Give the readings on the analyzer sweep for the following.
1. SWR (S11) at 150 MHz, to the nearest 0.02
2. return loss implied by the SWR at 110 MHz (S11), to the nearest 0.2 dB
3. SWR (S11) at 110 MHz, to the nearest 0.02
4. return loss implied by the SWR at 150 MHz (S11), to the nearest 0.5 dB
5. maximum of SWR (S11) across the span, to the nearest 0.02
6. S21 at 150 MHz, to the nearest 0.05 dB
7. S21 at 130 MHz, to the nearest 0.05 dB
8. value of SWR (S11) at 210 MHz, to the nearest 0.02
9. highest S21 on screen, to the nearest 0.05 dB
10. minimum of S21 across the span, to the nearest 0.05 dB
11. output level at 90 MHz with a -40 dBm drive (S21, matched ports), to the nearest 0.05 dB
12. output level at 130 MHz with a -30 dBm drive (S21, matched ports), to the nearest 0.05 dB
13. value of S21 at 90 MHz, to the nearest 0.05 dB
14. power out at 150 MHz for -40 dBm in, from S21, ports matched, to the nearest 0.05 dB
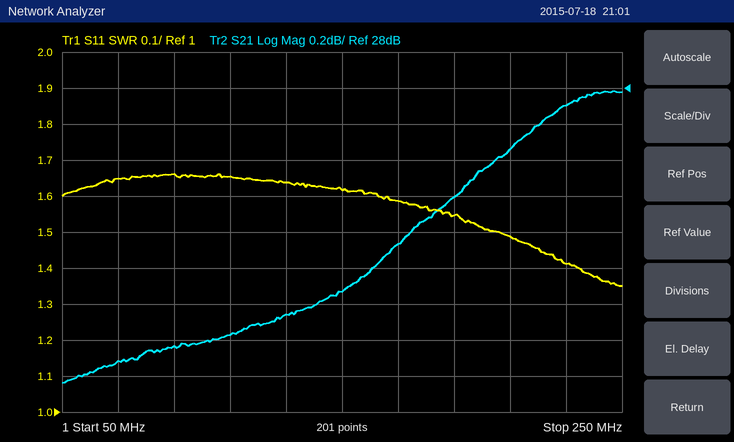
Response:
1.62
12.2 dB
1.66
12.5 dB
1.66
26.85 dB
26.75 dB
1.48
28.00 dB
26.35 dB
-13.45 dBm
-3.25 dBm
26.55 dB
-13.15 dBm
